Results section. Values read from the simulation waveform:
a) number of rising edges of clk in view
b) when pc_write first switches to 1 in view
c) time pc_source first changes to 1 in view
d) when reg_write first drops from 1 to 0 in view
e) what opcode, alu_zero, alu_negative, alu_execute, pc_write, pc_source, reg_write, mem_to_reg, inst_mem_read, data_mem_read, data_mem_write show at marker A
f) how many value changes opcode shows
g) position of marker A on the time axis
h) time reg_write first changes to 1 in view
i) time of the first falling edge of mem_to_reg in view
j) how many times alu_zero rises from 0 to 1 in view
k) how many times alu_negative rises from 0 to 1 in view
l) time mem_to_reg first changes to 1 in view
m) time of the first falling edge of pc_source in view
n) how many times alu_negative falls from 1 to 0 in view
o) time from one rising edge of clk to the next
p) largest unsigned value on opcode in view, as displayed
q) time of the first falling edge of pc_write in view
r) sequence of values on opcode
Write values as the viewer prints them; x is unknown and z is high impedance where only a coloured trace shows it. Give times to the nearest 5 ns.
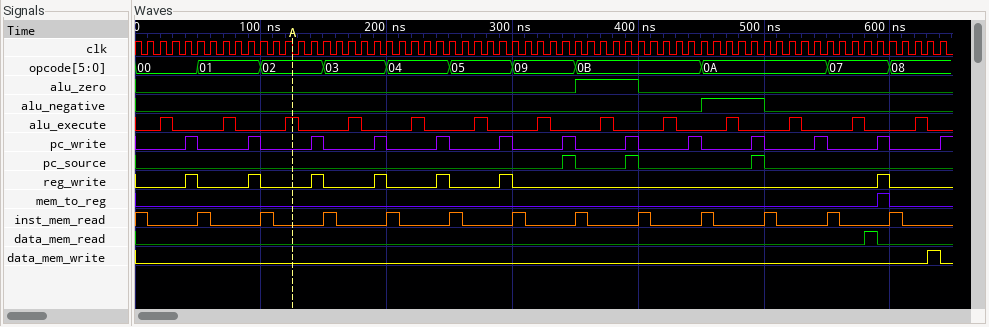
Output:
64
40 ns
340 ns
50 ns
opcode=02, alu_zero=0, alu_negative=0, alu_execute=1, pc_write=0, pc_source=0, reg_write=0, mem_to_reg=0, inst_mem_read=0, data_mem_read=0, data_mem_write=0
10
125 ns
40 ns
600 ns
1
1
590 ns
350 ns
1
10 ns
0B
50 ns
00, 01, 02, 03, 04, 05, 09, 0B, 0A, 07, 08
